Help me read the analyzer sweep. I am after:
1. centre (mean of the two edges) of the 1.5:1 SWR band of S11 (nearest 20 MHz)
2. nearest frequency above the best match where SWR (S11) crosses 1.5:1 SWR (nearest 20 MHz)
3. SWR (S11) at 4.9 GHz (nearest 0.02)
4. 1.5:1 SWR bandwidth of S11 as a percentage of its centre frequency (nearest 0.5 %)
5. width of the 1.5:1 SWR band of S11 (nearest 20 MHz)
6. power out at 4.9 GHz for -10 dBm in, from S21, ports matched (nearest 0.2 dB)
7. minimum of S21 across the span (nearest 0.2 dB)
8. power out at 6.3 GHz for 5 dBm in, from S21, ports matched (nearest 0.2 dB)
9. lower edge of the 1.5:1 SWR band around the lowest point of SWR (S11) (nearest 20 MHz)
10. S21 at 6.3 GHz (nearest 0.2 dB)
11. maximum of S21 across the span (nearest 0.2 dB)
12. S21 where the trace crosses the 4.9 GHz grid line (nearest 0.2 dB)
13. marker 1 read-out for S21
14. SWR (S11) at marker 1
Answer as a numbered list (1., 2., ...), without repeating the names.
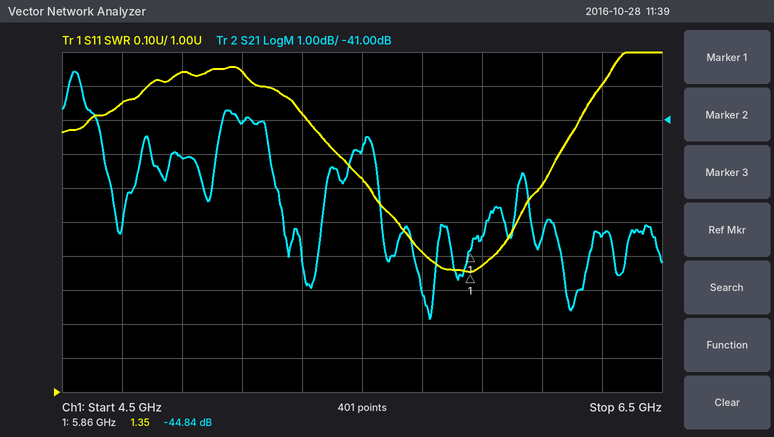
1. 5.82 GHz
2. 6.02 GHz
3. 1.94
4. 7.0 %
5. 400 MHz
6. -52.2 dBm
7. -46.8 dB
8. -39.4 dBm
9. 5.62 GHz
10. -44.4 dB
11. -39.6 dB
12. -42.2 dB
13. -44.84 dB
14. 1.35
